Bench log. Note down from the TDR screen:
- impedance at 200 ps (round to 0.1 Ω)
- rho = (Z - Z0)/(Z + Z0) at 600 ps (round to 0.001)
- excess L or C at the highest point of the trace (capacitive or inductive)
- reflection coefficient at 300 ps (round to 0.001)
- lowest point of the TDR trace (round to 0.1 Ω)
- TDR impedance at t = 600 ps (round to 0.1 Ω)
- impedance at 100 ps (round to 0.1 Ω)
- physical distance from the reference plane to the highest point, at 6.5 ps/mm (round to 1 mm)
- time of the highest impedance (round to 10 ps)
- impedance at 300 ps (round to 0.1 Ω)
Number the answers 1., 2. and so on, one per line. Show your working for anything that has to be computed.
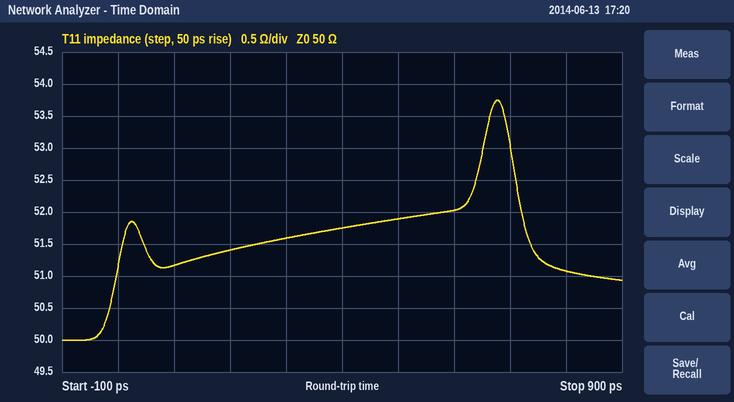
1. 51.4 Ω
2. (52 − 50)/(52 + 50) ≈ +0.020
3. inductive
4. (51.6 − 50)/(51.6 + 50) ≈ +0.016
5. 50.0 Ω
6. 52.0 Ω
7. 51.2 Ω
8. 680 ps / 2 / 6.5 ps/mm ≈ 52 mm
9. 680 ps
10. 51.6 Ω
